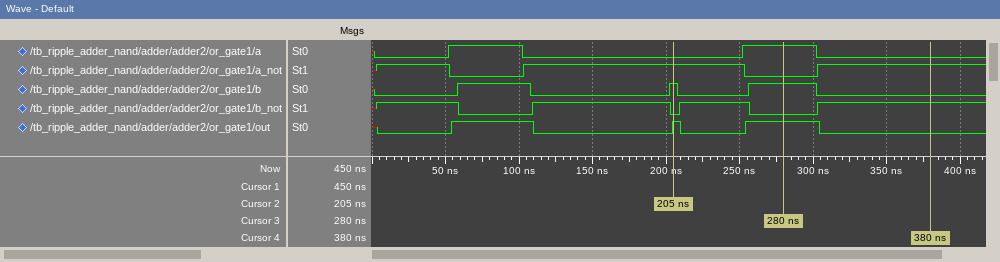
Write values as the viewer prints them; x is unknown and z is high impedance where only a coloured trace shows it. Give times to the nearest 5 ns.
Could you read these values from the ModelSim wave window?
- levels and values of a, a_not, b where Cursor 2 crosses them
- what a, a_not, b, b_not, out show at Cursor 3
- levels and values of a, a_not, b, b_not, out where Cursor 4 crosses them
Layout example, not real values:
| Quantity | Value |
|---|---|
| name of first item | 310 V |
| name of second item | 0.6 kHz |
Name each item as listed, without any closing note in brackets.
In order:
| Quantity | Value |
|---|---|
| levels and values of a, a_not, b where Cursor 2 crosses them | a=0, a_not=1, b=1 |
| what a, a_not, b, b_not, out show at Cursor 3 | a=1, a_not=0, b=1, b_not=0, out=1 |
| levels and values of a, a_not, b, b_not, out where Cursor 4 crosses them | a=0, a_not=1, b=0, b_not=1, out=0 |
